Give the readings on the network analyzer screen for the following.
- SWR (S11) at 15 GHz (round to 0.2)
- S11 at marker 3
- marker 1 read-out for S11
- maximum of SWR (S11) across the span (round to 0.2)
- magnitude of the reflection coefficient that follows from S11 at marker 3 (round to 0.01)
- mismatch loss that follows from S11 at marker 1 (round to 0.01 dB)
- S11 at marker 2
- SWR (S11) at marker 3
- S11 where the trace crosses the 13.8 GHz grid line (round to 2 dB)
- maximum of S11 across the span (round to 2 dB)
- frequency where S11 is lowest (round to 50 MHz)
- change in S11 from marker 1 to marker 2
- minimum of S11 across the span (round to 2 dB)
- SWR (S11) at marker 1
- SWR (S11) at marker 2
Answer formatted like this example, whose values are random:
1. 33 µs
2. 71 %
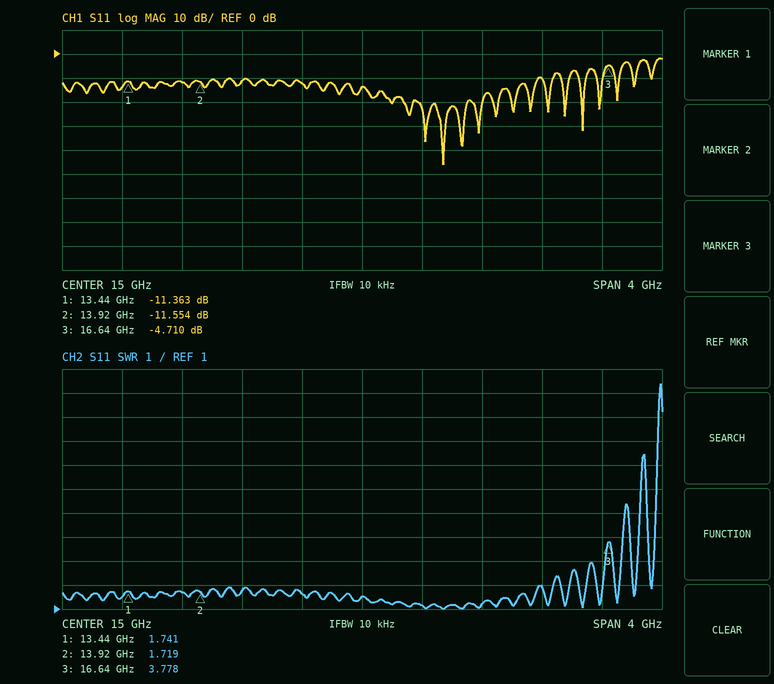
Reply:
1. 1.6
2. -4.710 dB
3. -11.363 dB
4. 10.4
5. 0.58
6. 0.33 dB
7. -11.554 dB
8. 3.778
9. -12 dB
10. -2 dB
11. 15.55 GHz
12. -0.191 dB
13. -46 dB
14. 1.741
15. 1.719
